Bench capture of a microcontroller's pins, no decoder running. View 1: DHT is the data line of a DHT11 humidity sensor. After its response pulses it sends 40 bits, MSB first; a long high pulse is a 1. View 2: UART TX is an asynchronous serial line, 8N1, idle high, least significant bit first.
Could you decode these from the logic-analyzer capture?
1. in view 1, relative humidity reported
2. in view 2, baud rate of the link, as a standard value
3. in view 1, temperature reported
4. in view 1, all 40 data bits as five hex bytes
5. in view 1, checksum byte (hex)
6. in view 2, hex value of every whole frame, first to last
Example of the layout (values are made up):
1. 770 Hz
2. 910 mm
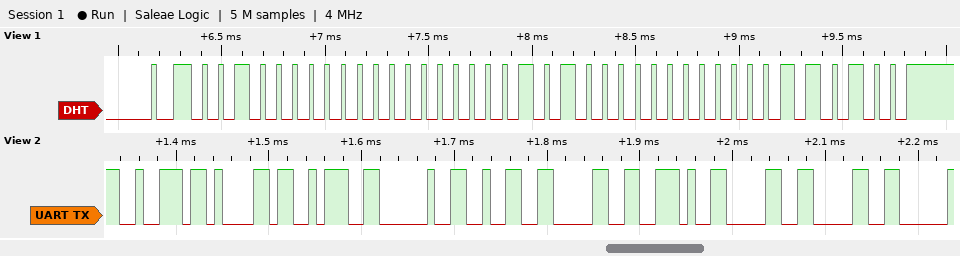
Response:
1. 32 %
2. 115200 baud
3. 20.0 °C
4. 20 00 14 00 34
5. 0x34
6. 0x72 0x61 0x3A 0x20 0x32 0x30 0x2E 0x30 0x30
